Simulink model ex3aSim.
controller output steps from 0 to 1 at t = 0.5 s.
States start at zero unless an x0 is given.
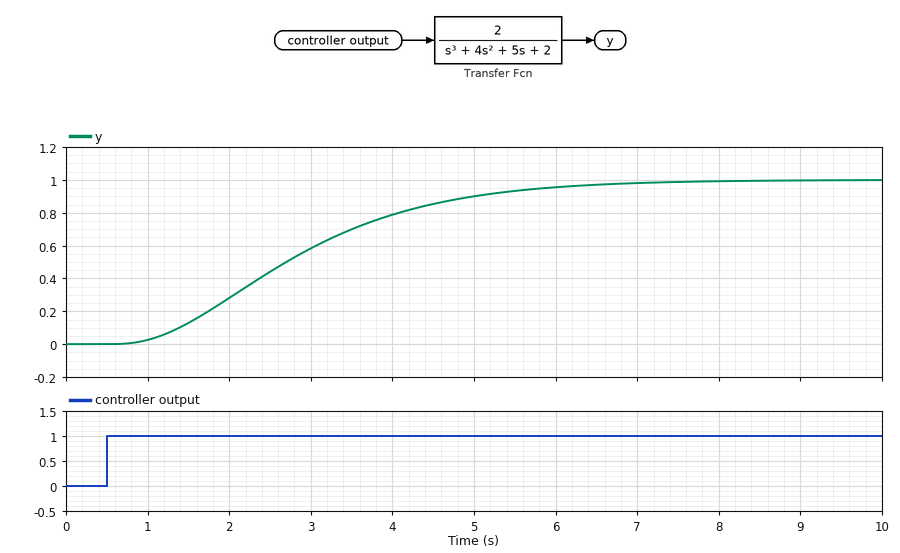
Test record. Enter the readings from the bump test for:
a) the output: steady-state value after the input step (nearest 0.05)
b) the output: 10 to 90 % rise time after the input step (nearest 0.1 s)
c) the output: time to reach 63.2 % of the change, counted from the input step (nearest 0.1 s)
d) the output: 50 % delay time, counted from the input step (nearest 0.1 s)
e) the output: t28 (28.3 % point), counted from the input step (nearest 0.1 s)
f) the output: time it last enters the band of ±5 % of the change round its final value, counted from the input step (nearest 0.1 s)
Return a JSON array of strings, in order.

["1.00", "3.6 s", "2.7 s", "2.2 s", "1.5 s", "5.4 s"]
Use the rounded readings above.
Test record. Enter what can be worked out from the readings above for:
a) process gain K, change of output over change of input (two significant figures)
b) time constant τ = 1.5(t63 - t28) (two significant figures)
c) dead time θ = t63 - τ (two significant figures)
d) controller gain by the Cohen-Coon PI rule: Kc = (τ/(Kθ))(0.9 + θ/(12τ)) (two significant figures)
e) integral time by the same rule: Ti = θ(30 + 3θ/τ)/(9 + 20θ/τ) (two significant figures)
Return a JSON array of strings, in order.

["1.0", "1.8 s", "0.90 s", "1.9", "1.5 s"]
